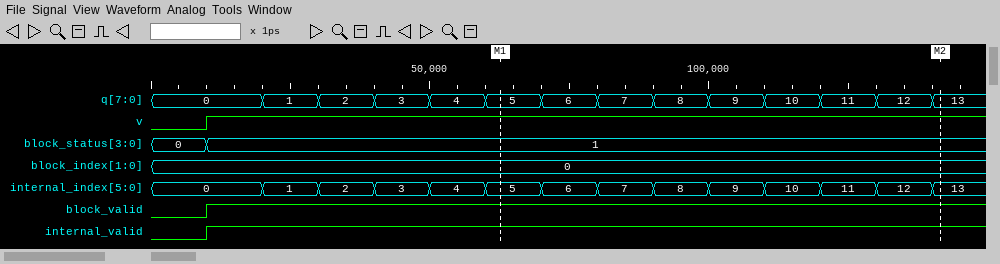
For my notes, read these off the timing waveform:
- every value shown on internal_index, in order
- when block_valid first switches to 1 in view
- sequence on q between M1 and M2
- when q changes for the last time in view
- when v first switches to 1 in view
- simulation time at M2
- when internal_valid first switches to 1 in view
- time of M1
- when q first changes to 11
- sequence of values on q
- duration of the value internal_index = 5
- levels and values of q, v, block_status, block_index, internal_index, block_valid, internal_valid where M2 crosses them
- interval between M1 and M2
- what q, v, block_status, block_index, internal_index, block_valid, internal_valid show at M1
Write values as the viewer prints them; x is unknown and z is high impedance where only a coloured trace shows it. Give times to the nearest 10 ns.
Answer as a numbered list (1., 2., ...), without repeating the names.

1. 0, 1, 2, 3, 4, 5, 6, 7, 8, 9, 10, 11, 12, 13
2. 10 ns
3. 5, 6, 7, 8, 9, 10, 11, 12, 13
4. 140 ns
5. 10 ns
6. 140 ns
7. 10 ns
8. 60 ns
9. 120 ns
10. 0, 1, 2, 3, 4, 5, 6, 7, 8, 9, 10, 11, 12, 13
11. 10 ns
12. q=13, v=1, block_status=1, block_index=0, internal_index=13, block_valid=1, internal_valid=1
13. 80 ns
14. q=5, v=1, block_status=1, block_index=0, internal_index=5, block_valid=1, internal_valid=1
